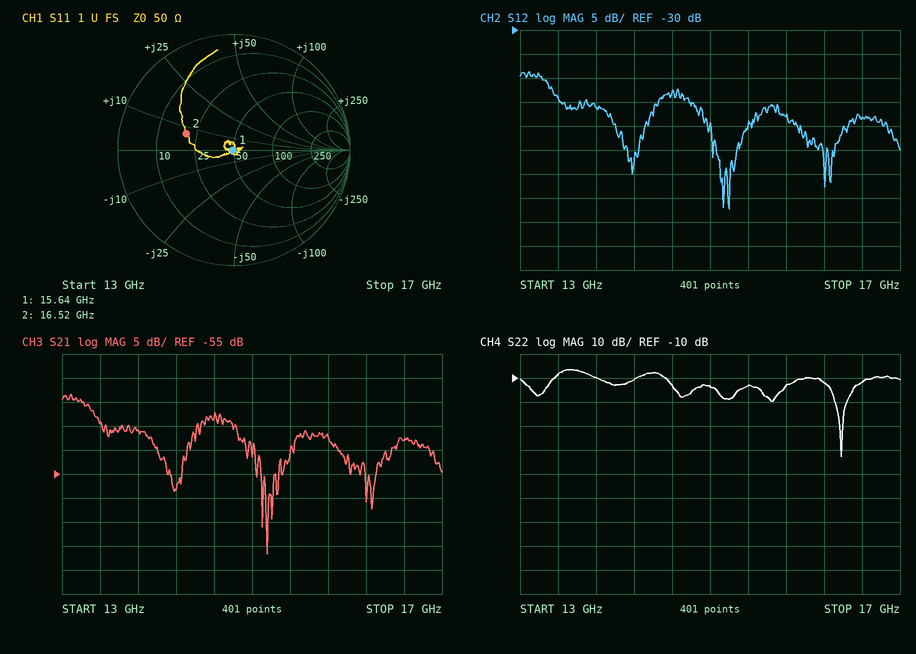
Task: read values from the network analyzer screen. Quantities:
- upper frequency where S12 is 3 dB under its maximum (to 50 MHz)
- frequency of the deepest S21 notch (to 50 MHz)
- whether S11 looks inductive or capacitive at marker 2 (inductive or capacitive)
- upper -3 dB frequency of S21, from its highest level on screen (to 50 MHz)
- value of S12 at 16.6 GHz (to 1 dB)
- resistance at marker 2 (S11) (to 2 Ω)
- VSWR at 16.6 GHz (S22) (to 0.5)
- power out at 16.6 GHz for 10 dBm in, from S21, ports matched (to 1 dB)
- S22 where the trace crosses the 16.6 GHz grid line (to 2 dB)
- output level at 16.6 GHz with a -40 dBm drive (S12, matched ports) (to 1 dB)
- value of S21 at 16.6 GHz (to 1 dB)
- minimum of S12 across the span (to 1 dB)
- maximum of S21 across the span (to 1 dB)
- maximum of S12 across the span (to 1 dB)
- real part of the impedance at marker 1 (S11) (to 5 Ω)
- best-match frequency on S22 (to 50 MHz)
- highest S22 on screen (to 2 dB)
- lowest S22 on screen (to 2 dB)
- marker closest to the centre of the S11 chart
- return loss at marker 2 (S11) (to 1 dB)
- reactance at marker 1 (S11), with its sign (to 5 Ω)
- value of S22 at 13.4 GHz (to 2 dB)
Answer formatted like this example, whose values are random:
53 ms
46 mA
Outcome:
13.30 GHz
15.15 GHz
inductive
13.30 GHz
-48 dB
20 Ω
1.5
-38 dBm
-12 dB
-88 dBm
-48 dB
-67 dB
-38 dB
-39 dB
50 Ω
16.40 GHz
-6 dB
-42 dB
marker 1
7 dB
0 Ω
-8 dB
